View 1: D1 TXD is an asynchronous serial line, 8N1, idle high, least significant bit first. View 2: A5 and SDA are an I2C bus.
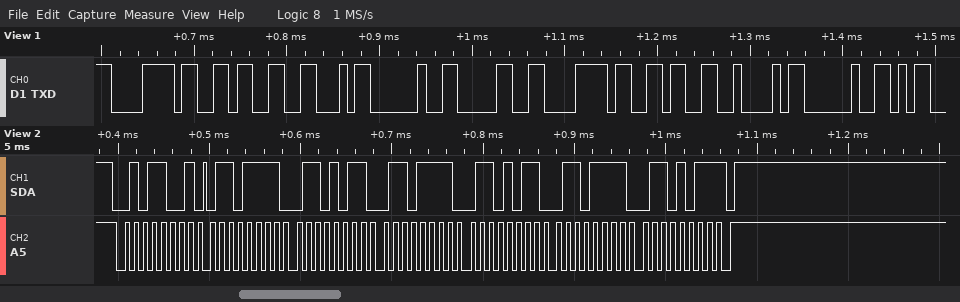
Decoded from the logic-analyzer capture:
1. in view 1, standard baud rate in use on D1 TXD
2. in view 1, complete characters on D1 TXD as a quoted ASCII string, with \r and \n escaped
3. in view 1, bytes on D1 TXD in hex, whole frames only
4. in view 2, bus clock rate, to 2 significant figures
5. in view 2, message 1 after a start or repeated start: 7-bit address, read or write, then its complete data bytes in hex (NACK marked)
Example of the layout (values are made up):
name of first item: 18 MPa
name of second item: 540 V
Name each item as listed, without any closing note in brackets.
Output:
in view 1, standard baud rate in use on D1 TXD: 115200 baud
in view 1, complete characters on D1 TXD as a quoted ASCII string, with \r and \n escaped: "x6F 0x6B "
in view 1, bytes on D1 TXD in hex, whole frames only: 0x78 0x36 0x46 0x20 0x30 0x78 0x36 0x42 0x20
in view 2, bus clock rate, to 2 significant figures: 100 kHz
in view 2, message 1 after a start or repeated start: 7-bit address, read or write, then its complete data bytes in hex: 0x2C read: 6F 6B 6F 6B 6F 6B NACK
